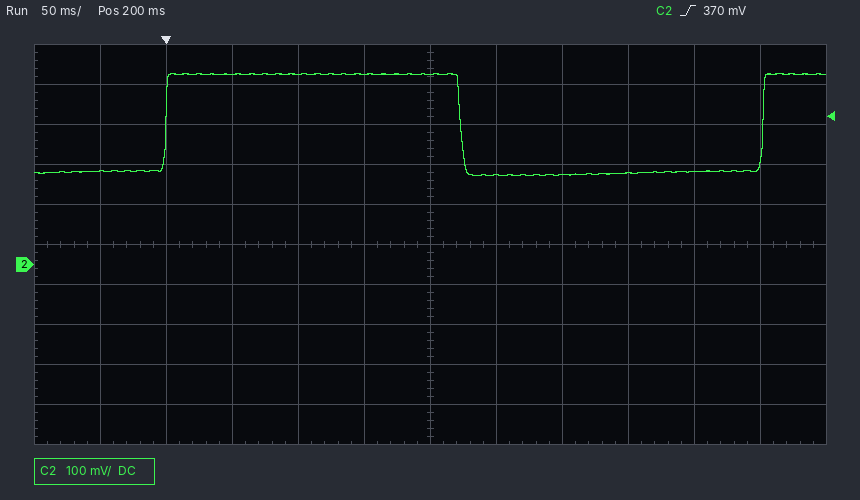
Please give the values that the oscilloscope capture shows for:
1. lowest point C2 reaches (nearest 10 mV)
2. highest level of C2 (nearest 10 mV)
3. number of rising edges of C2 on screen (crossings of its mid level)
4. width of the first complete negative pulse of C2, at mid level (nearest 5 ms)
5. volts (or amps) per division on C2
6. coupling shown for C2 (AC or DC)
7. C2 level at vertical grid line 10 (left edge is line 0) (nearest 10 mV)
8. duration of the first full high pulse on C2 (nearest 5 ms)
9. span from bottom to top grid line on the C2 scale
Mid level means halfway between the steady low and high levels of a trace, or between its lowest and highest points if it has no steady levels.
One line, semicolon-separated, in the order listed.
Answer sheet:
220 mV; 480 mV; 2; 230 ms; 100 mV; DC; 230 mV; 225 ms; 1 V
